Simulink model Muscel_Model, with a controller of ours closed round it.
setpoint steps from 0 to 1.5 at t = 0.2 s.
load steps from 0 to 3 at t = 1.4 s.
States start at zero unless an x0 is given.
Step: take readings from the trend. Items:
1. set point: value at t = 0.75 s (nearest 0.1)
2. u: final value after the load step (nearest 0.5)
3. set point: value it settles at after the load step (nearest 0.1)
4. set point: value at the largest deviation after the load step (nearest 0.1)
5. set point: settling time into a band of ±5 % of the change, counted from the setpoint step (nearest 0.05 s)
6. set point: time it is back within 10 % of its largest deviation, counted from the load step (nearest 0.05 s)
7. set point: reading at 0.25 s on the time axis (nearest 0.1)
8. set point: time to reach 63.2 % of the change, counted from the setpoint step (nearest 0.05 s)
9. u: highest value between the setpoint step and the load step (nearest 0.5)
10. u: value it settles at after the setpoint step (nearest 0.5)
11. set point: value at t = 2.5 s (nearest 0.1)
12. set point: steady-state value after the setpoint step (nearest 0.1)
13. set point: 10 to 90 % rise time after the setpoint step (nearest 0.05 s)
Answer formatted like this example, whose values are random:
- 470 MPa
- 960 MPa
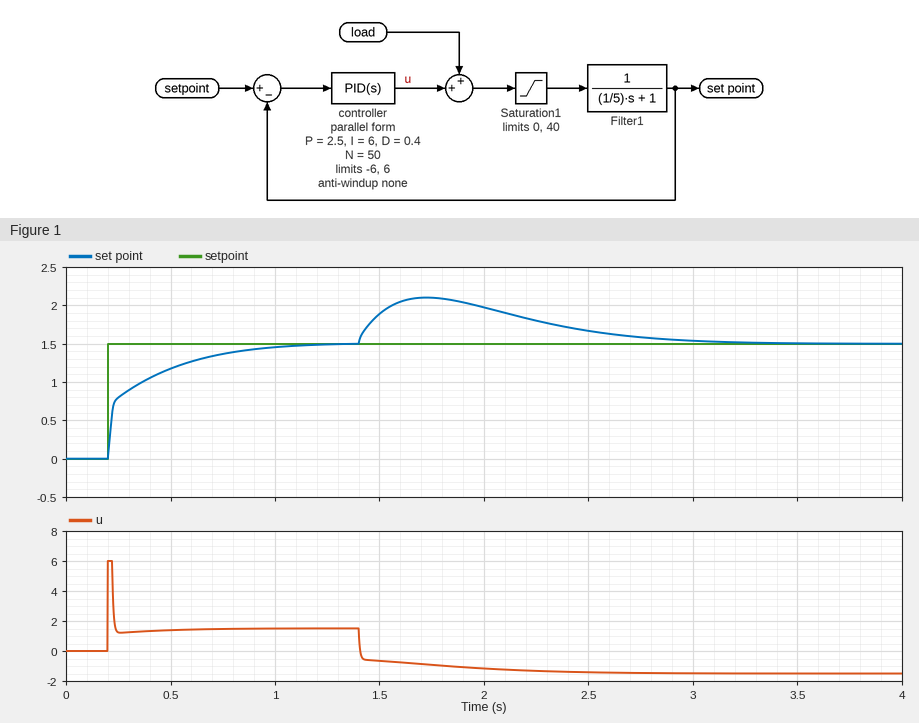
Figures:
- 1.4
- -1.5
- 1.5
- 2.1
- 0.70 s
- 1.45 s
- 0.8
- 0.15 s
- 6.0
- 1.5
- 1.7
- 1.5
- 0.50 s
